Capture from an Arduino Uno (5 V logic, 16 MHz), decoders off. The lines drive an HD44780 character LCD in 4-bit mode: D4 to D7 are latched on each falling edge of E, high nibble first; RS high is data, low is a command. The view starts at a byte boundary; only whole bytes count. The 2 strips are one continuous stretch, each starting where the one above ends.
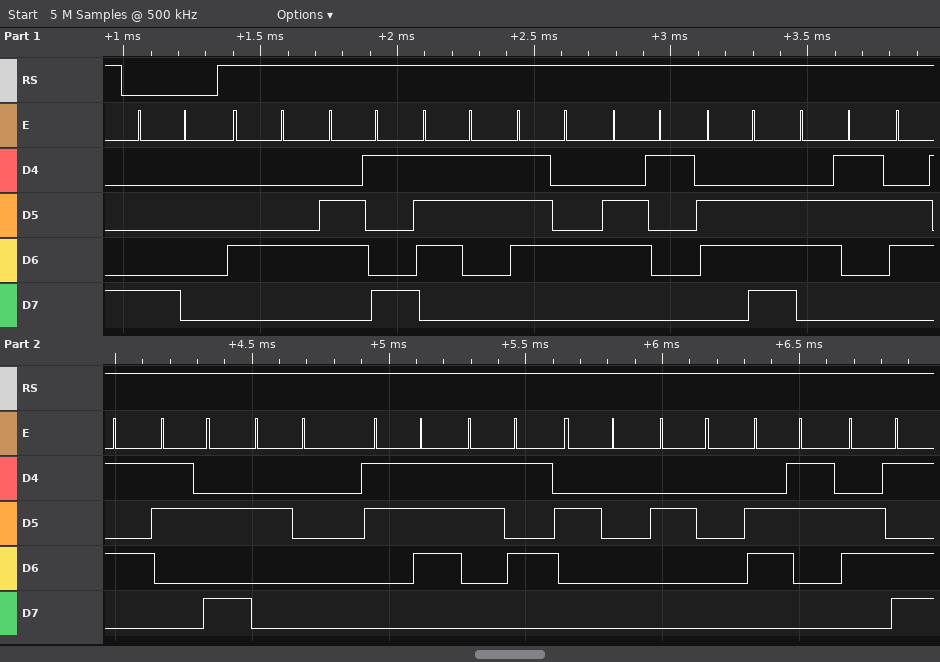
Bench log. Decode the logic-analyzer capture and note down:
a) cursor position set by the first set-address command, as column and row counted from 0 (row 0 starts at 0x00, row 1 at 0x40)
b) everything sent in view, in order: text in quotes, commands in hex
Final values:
column 0, row 0
0x80 "Distance: 75  cm"
